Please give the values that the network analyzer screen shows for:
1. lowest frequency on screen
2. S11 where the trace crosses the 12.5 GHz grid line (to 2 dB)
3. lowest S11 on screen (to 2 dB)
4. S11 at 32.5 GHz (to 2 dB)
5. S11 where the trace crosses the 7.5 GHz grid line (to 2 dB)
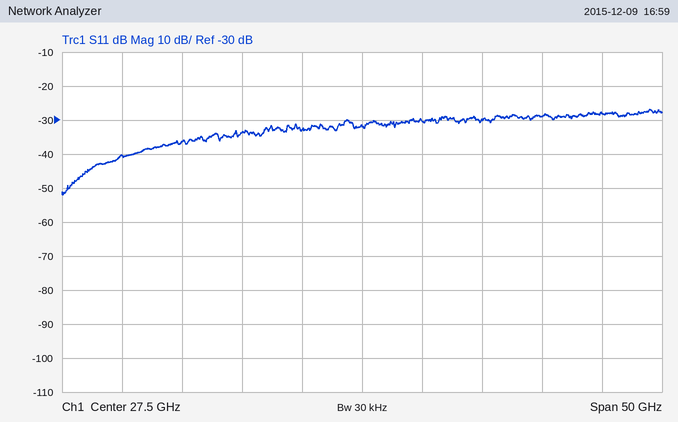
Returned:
2.5 GHz
-36 dB
-52 dB
-30 dB
-40 dB
